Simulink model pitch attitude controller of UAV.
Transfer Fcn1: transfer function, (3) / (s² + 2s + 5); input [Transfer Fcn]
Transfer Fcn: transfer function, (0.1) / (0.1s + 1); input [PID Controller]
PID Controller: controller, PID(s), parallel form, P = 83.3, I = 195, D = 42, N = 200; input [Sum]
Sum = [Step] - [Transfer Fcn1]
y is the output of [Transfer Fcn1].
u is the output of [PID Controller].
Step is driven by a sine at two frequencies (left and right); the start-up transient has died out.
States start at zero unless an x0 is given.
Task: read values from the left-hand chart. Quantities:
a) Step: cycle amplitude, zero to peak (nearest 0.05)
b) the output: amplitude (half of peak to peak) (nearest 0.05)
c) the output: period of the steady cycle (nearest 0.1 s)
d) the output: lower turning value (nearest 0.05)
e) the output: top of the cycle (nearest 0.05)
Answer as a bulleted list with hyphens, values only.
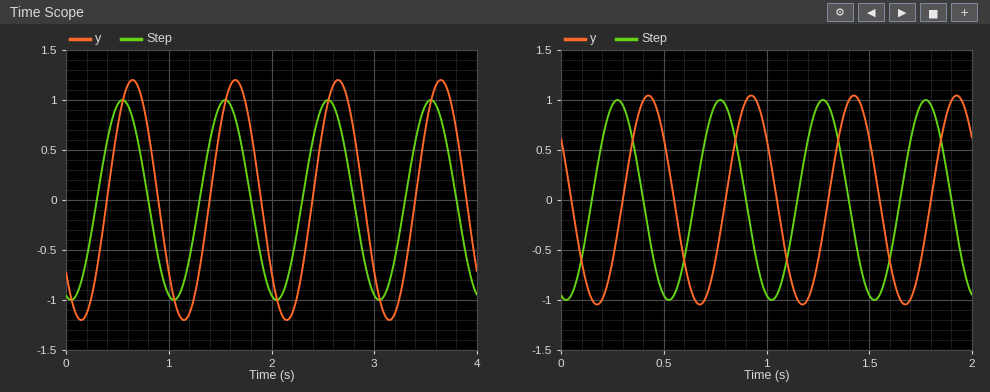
- 1.00
- 1.20
- 1.0 s
- -1.20
- 1.20
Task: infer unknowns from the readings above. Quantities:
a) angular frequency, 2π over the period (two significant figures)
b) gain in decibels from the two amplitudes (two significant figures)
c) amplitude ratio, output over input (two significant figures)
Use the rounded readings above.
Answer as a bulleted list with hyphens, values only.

- 6.3 rad/s
- 1.6 dB
- 1.2
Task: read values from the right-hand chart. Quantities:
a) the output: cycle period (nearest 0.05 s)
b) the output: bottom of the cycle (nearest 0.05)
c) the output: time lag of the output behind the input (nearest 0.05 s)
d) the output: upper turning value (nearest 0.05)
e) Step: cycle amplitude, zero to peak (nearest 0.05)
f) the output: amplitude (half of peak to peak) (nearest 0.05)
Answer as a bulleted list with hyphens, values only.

- 0.50 s
- -1.05
- 0.15 s
- 1.05
- 1.00
- 1.05
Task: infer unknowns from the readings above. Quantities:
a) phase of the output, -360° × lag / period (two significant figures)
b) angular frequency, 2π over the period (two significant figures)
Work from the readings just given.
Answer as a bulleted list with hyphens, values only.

- -110°
- 13 rad/s
